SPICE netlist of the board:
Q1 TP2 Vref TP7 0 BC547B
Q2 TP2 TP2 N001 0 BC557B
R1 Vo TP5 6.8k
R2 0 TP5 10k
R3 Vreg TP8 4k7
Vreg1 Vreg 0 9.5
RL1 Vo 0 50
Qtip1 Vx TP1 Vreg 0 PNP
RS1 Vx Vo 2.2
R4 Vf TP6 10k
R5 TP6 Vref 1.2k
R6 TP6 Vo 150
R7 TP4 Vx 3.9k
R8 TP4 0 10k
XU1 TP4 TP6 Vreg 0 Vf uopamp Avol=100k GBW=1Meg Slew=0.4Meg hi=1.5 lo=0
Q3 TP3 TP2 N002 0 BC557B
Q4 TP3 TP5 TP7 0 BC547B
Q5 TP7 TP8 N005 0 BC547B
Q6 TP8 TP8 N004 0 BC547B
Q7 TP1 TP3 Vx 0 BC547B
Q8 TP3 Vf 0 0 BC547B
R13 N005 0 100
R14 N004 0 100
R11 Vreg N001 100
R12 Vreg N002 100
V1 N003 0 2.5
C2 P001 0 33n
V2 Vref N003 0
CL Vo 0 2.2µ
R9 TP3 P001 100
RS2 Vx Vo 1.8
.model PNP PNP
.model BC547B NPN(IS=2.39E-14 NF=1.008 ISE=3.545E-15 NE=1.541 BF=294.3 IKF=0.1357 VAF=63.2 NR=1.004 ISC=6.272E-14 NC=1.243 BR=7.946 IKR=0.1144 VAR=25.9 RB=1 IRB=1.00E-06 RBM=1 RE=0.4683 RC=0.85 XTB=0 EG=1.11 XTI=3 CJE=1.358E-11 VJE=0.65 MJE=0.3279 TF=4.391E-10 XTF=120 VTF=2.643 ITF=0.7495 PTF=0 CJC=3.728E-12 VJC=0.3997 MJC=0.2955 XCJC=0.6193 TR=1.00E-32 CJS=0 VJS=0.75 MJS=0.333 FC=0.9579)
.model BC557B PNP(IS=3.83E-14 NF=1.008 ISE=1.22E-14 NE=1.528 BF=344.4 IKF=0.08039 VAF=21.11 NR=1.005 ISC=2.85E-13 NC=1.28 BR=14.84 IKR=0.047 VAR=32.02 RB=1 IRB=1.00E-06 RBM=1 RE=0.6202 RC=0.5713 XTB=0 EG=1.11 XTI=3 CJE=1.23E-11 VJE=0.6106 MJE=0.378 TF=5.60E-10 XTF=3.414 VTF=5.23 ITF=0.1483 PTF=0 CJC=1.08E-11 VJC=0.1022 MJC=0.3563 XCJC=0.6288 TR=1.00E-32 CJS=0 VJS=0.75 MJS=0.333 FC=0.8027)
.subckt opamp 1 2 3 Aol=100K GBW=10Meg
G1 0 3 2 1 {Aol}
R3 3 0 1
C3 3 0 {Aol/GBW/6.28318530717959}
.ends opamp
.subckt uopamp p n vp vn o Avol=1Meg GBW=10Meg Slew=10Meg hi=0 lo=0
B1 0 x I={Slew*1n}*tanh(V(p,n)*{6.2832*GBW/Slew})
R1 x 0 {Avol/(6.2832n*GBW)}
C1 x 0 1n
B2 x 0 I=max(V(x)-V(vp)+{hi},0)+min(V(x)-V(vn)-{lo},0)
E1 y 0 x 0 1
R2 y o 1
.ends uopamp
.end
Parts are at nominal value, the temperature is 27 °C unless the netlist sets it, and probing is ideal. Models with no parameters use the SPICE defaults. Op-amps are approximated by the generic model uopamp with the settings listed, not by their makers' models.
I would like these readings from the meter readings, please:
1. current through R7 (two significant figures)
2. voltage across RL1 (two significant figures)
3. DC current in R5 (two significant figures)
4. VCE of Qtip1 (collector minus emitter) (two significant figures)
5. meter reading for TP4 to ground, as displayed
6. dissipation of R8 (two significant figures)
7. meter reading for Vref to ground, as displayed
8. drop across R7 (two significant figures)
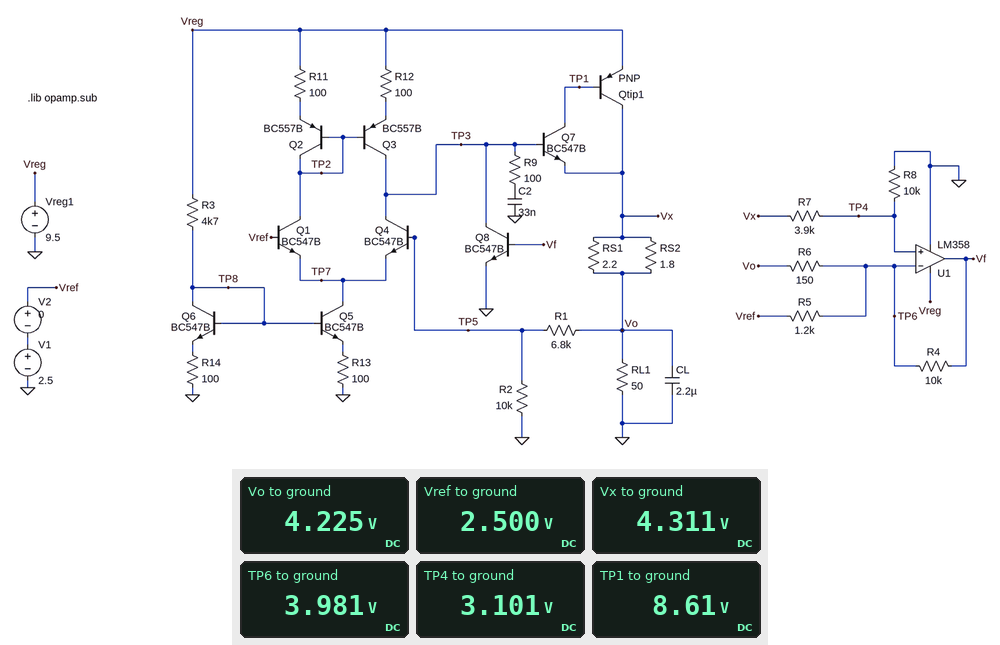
310 µA
4.2 V
1.2 mA
-5.2 V
3.101 V
960 µW
2.500 V
1.2 V
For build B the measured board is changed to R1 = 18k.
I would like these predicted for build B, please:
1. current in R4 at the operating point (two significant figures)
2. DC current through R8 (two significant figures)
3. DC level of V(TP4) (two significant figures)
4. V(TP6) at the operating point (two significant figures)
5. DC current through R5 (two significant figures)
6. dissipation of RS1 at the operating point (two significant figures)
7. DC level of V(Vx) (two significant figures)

650 µA
520 µA
5.2 V
6.5 V
3.3 mA
9.4 mW
7.2 V
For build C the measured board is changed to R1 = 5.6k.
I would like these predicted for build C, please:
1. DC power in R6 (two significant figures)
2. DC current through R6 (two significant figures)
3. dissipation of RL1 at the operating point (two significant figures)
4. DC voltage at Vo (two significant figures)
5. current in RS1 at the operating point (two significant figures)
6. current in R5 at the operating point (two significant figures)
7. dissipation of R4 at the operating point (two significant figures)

290 µW
1.4 mA
310 mW
3.9 V
36 mA
1.0 mA
1.4 mW
